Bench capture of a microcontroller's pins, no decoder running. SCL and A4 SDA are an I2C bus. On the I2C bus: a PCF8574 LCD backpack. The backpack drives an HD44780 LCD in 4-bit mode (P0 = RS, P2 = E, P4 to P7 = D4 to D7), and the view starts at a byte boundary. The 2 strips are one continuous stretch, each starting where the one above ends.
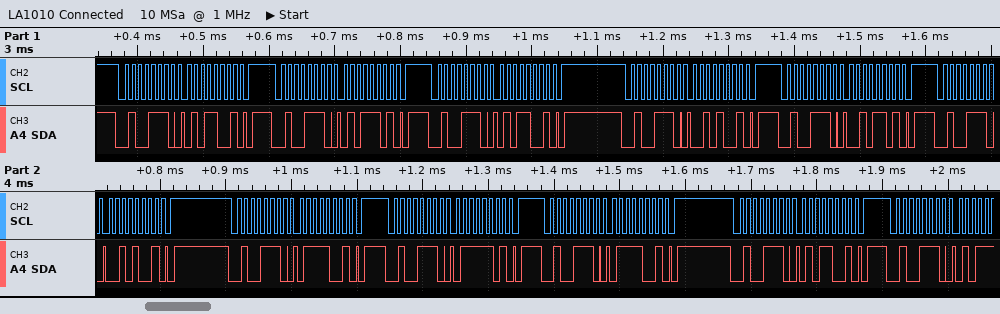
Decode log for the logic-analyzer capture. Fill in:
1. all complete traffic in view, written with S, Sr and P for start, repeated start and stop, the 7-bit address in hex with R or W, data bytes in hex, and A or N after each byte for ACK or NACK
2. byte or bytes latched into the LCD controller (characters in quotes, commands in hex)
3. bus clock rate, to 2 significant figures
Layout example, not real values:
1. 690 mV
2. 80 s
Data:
1. S 27W A 59 A P S 27W A 5D A P S 27W A 59 A P S 27W A 29 A P S 27W A 2D A P S 27W A 29 A P S 27W A 79 A P S 27W A 7D A P S 27W A 79 A P S 27W A 59 A P S 27W A
2. 'R'
3. 100 kHz
